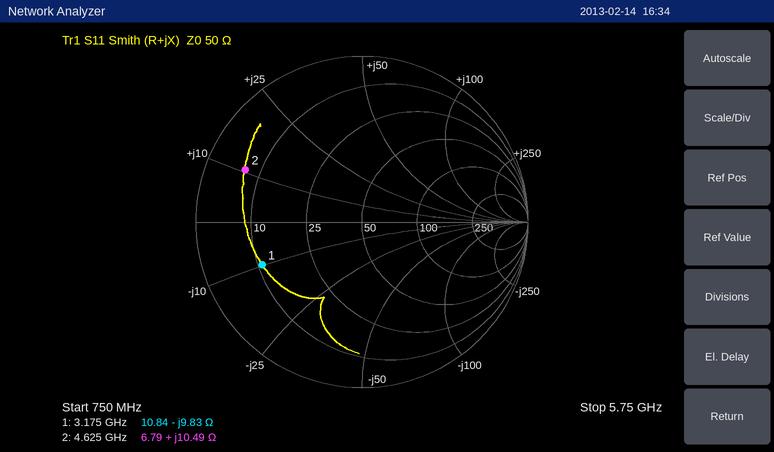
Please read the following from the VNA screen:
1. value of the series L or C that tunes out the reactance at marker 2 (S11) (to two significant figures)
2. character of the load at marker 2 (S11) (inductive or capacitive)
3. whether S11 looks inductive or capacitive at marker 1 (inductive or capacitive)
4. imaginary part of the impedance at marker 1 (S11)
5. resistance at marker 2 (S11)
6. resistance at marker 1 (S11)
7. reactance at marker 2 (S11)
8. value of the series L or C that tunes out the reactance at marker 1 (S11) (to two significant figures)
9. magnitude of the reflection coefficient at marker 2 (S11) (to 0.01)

3.3 pF
inductive
capacitive
-9.83 Ω
6.79 Ω
10.84 Ω
+10.49 Ω
490 pH
0.77
